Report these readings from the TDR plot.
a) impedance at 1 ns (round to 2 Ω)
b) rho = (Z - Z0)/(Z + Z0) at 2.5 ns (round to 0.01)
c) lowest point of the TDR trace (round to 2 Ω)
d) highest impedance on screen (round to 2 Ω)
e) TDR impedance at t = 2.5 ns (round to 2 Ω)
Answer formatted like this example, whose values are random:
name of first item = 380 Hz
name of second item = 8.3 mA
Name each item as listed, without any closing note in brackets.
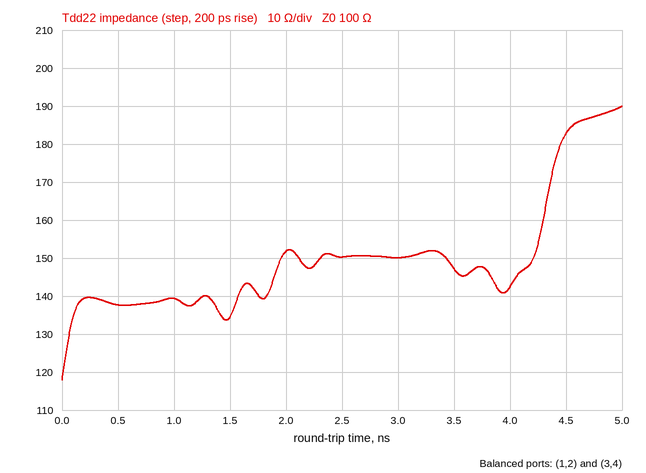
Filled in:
impedance at 1 ns = 140 Ω
rho = (Z - Z0)/(Z + Z0) at 2.5 ns = +0.20
lowest point of the TDR trace = 118 Ω
highest impedance on screen = 190 Ω
TDR impedance at t = 2.5 ns = 150 Ω
